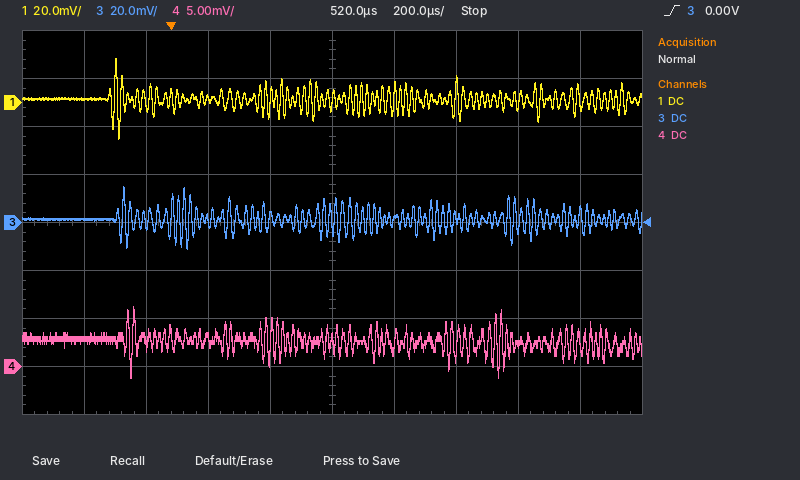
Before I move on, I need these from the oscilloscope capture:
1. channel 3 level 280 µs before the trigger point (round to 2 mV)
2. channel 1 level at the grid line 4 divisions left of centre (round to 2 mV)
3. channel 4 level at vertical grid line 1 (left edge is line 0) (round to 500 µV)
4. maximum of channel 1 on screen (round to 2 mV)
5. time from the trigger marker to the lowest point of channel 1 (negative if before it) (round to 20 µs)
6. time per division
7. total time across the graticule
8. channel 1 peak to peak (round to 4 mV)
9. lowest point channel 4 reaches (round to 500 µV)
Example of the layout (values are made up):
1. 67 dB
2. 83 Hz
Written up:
1. 2 mV
2. 2 mV
3. 3.0 mV
4. 18 mV
5. -160 µs
6. 200 µs
7. 2 ms
8. 32 mV
9. -1.0 mV
